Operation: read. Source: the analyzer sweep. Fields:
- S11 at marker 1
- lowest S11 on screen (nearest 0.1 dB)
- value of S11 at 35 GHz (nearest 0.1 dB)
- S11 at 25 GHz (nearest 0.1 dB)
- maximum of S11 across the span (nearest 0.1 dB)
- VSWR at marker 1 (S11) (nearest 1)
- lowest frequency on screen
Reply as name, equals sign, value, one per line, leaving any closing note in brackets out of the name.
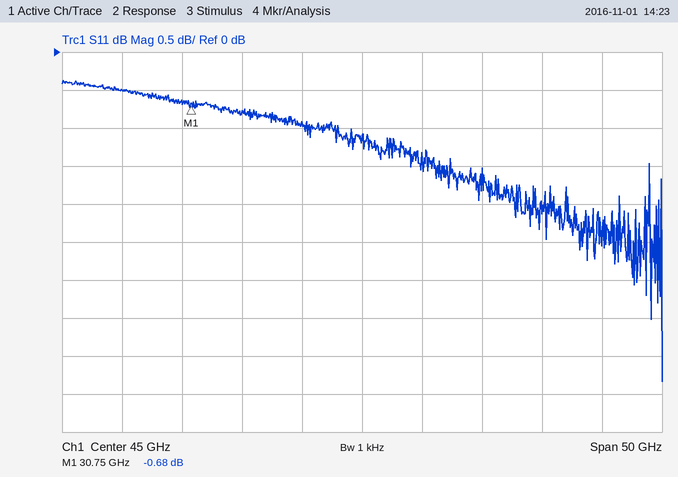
S11 at marker 1 = -0.68 dB
lowest S11 on screen = -4.3 dB
value of S11 at 35 GHz = -0.8 dB
S11 at 25 GHz = -0.5 dB
maximum of S11 across the span = -0.4 dB
VSWR at marker 1 (S11) = 26
lowest frequency on screen = 20 GHz
